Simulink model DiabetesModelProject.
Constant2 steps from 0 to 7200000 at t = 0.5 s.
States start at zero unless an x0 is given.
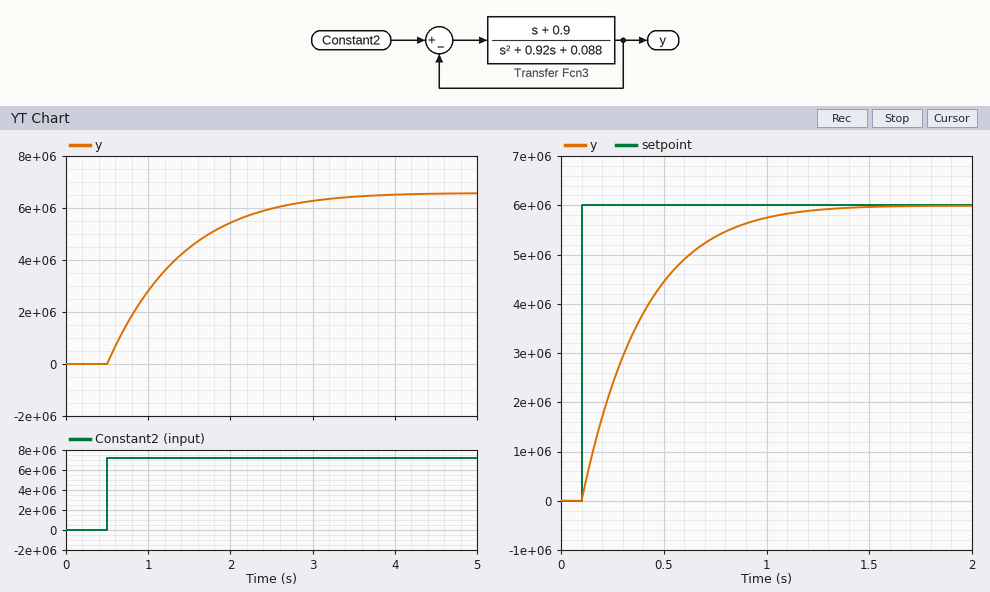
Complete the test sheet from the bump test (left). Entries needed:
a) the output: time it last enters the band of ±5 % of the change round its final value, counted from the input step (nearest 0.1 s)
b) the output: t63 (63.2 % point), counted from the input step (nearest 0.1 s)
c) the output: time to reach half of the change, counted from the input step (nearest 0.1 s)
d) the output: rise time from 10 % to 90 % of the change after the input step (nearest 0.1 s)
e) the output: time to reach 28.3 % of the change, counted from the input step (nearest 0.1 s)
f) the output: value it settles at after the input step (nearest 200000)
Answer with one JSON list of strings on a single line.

["2.4 s", "0.9 s", "0.6 s", "1.8 s", "0.3 s", "6600000"]
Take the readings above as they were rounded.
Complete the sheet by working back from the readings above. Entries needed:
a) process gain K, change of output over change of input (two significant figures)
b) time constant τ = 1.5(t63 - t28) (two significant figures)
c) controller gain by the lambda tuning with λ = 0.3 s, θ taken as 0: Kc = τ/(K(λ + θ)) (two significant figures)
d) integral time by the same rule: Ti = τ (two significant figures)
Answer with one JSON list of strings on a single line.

["0.92", "0.90 s", "3.3", "0.90 s"]
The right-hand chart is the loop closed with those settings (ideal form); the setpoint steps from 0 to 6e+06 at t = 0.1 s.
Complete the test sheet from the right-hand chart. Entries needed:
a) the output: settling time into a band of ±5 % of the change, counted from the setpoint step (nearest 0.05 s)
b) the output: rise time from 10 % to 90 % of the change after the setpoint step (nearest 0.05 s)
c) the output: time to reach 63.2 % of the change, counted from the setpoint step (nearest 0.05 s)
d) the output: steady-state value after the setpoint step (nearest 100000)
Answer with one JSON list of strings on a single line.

["0.85 s", "0.65 s", "0.30 s", "6000000"]
